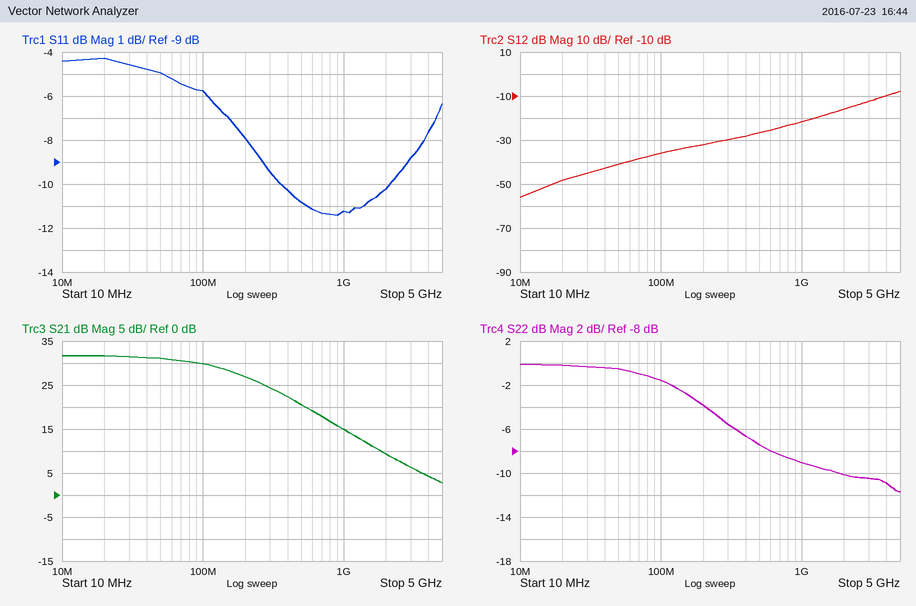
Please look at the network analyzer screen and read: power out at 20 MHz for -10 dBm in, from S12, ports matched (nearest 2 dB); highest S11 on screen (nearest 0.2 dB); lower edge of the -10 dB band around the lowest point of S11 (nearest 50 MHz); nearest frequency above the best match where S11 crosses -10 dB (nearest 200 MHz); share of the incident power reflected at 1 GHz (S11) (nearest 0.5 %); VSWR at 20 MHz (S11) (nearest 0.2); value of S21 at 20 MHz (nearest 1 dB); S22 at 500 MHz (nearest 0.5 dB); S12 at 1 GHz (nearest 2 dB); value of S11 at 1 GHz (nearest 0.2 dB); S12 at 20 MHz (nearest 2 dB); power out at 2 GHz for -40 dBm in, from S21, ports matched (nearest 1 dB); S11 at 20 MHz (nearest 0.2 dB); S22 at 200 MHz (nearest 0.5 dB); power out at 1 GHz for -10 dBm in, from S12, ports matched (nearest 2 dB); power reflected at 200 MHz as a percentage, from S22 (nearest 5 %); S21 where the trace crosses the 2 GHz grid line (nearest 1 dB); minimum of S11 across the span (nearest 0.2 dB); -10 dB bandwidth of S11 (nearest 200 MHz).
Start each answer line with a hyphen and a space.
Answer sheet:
- -58 dBm
- -4.2 dB
- 350 MHz
- 2.2 GHz
- 7.5 %
- 4.2
- 32 dB
- -7.5 dB
- -22 dB
- -11.2 dB
- -48 dB
- -31 dBm
- -4.2 dB
- -4.0 dB
- -32 dBm
- 40 %
- 9 dB
- -11.4 dB
- 1.8 GHz
